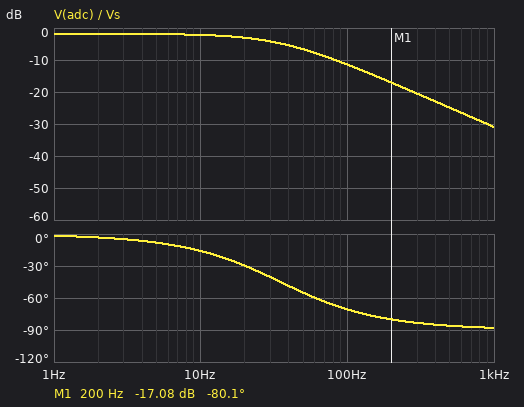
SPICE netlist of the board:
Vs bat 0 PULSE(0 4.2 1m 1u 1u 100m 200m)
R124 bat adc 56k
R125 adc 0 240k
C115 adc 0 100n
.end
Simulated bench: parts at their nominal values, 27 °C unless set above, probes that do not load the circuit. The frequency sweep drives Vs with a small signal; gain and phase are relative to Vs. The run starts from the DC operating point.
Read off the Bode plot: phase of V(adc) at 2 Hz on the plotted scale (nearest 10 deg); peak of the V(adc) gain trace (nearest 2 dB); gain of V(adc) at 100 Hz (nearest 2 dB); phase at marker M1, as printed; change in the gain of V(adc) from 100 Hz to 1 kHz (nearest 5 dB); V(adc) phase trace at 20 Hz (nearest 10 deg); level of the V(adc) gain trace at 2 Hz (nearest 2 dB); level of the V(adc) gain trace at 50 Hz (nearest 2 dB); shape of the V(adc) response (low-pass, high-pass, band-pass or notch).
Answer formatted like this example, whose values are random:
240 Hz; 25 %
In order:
0 deg; -2 dB; -12 dB; -80.1 deg; -20 dB; -30 deg; -2 dB; -6 dB; low-pass
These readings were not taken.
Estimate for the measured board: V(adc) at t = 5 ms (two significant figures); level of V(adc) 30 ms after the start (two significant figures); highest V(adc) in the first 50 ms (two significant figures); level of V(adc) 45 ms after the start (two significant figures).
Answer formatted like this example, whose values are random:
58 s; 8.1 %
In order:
2.0 V; 3.4 V; 3.4 V; 3.4 V
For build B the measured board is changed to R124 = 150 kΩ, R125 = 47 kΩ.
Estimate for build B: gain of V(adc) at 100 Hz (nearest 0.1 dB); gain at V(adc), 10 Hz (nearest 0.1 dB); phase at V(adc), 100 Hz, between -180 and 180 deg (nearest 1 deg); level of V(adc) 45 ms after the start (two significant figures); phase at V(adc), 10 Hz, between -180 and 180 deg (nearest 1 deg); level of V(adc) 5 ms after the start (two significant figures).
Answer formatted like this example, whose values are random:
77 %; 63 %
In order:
-20.3 dB; -12.7 dB; -66 deg; 1.0 V; -13 deg; 670 mV
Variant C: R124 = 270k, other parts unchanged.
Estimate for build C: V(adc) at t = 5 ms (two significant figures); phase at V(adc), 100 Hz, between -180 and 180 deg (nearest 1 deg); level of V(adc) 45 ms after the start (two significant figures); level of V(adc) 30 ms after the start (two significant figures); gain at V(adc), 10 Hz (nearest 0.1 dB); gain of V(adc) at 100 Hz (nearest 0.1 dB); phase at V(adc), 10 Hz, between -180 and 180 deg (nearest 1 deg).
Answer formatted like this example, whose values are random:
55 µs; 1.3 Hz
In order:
530 mV; -83 deg; 1.9 V; 1.8 V; -8.7 dB; -24.7 dB; -39 deg
